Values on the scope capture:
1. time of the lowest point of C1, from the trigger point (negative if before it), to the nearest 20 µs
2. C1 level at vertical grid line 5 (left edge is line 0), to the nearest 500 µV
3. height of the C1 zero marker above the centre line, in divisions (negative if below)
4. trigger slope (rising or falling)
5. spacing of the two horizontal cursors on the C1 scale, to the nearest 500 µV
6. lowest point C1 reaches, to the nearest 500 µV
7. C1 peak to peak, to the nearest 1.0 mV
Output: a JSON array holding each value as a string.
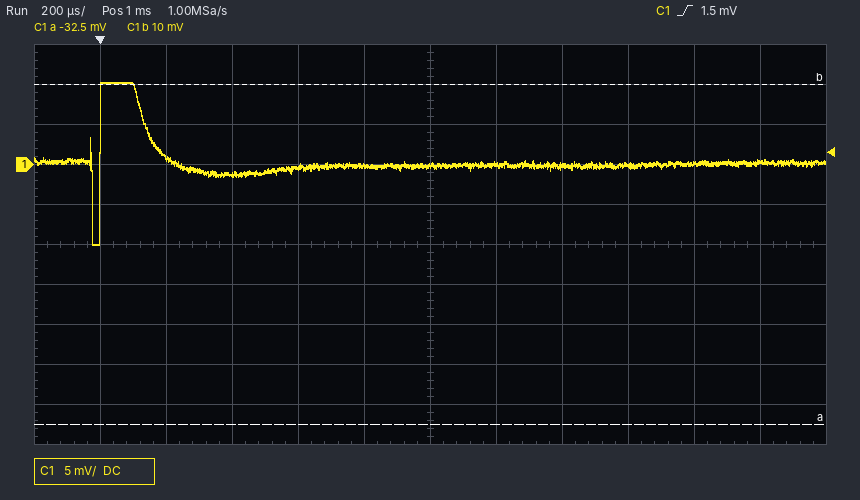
["-20 µs", "0.0 mV", "+2.0 div", "rising", "42.5 mV", "-10.0 mV", "20.0 mV"]
